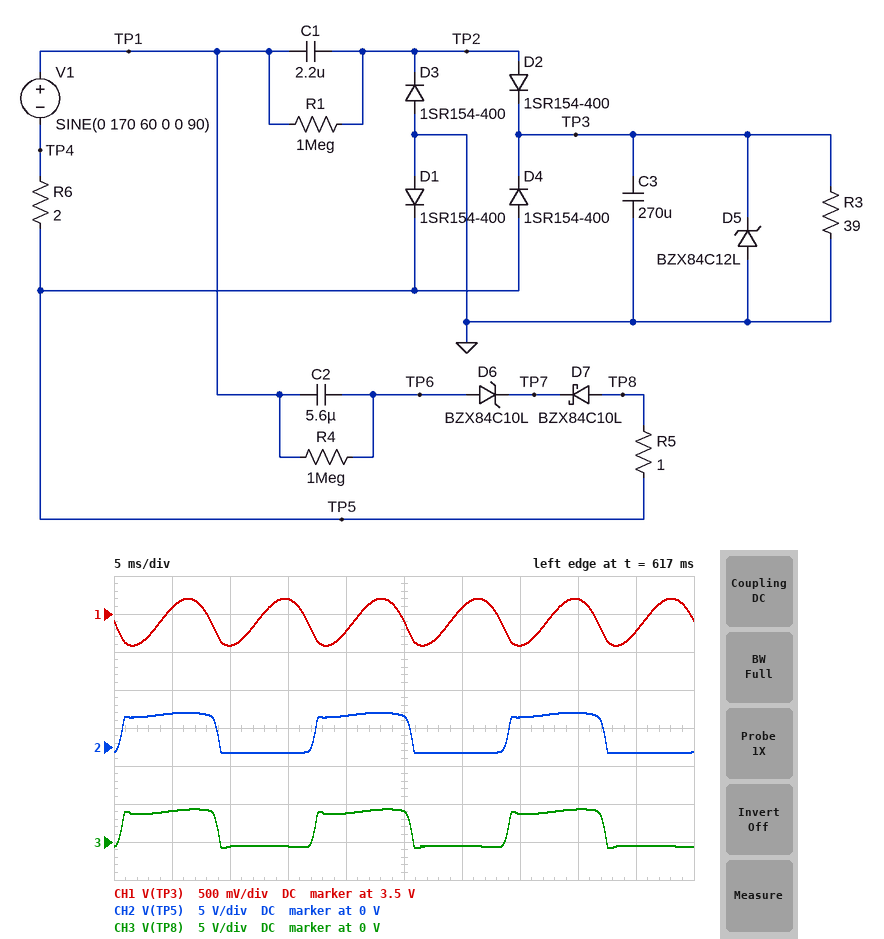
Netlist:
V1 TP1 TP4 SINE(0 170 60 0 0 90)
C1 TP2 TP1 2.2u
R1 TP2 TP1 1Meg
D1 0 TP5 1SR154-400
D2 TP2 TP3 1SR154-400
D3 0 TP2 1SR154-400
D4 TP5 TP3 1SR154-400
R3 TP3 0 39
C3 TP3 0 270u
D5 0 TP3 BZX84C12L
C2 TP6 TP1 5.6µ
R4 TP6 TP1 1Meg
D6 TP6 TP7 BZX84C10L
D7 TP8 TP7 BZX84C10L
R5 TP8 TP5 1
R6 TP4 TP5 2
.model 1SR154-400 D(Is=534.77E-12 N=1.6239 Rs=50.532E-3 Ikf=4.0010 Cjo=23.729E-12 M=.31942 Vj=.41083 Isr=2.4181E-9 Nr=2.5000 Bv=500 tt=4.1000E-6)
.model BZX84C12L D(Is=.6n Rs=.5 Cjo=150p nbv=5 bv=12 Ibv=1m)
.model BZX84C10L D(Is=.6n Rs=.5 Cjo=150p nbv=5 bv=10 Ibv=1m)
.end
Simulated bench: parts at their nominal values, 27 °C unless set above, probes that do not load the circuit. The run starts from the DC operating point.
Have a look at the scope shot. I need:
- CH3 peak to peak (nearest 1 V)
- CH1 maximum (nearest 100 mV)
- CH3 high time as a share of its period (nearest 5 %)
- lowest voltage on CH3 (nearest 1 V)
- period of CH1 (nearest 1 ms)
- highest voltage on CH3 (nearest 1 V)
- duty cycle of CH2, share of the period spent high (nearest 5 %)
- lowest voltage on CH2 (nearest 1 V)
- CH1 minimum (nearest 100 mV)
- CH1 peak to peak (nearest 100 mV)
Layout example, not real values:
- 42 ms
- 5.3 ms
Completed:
- 5 V
- 3.7 V
- 50 %
- -1 V
- 8 ms
- 4 V
- 50 %
- -1 V
- 3.1 V
- 600 mV
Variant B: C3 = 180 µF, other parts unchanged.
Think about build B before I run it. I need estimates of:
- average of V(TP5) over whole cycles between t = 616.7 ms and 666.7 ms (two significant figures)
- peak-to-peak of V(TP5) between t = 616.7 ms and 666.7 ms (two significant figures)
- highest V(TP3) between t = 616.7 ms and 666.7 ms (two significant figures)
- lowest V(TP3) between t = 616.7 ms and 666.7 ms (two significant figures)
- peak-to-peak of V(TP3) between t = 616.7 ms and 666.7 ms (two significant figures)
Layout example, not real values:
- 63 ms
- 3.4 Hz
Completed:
- 1.7 V
- 5.5 V
- 3.8 V
- 2.9 V
- 920 mV
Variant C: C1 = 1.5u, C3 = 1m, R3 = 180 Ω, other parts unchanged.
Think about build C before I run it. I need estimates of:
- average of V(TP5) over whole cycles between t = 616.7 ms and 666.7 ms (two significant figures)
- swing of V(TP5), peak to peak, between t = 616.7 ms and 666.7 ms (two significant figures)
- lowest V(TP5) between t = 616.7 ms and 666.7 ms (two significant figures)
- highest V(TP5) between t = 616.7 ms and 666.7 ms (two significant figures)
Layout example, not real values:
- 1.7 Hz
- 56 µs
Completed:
- 5.0 V
- 12 V
- -810 mV
- 11 V
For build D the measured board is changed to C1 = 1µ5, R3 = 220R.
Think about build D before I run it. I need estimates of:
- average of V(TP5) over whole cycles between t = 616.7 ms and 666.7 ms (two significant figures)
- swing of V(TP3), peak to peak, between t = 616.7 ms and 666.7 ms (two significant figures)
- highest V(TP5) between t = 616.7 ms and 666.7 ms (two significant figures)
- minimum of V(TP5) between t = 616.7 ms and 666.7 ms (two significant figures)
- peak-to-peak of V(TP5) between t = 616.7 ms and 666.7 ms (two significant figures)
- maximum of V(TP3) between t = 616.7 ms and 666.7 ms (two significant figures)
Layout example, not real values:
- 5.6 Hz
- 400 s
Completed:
- 6.0 V
- 480 mV
- 13 V
- -810 mV
- 14 V
- 12 V
